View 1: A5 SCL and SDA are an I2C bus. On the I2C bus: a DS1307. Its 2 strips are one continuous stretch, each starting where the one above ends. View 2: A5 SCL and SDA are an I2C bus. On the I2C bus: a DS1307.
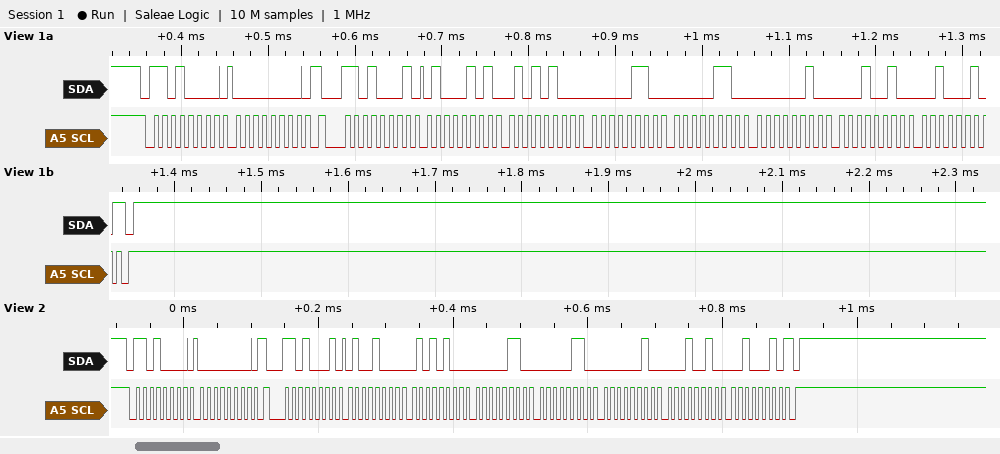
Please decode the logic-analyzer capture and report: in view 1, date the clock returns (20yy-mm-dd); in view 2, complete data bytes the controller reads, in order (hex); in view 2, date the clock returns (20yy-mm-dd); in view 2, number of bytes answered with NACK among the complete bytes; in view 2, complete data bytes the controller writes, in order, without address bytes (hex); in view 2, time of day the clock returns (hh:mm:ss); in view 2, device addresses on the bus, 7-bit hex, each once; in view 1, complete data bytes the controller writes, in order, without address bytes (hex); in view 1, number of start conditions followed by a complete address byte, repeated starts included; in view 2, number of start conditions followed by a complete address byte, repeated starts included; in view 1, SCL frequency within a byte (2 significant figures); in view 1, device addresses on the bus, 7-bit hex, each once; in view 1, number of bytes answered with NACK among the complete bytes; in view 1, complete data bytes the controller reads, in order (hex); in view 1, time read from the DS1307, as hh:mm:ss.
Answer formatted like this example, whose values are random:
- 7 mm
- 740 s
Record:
- 2022-12-02
- 48 54 06 06 02 12 22
- 2022-12-02
- 1
- 00
- 06:54:48
- 0x68
- 00
- 2
- 2
- 100 kHz
- 0x68
- 1
- 45 54 06 06 02 12 22
- 06:54:45
